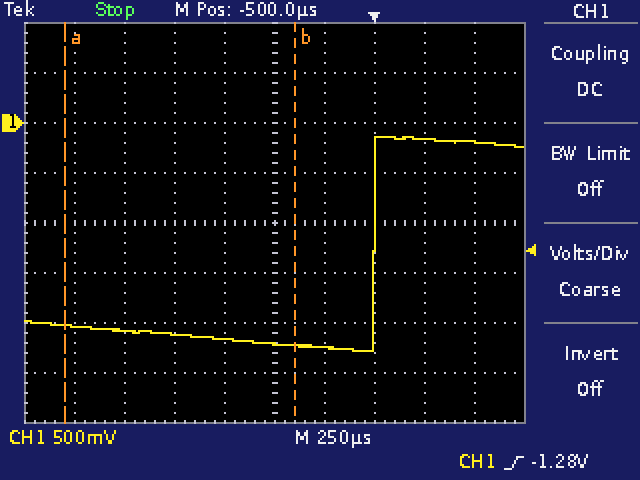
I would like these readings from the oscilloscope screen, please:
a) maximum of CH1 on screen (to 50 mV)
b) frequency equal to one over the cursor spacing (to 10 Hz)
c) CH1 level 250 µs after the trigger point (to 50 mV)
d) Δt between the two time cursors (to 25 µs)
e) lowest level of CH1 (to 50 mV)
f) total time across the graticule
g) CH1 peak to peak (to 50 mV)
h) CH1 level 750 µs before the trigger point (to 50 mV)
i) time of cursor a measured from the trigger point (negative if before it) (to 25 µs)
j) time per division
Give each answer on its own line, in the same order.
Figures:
-150 mV
870 Hz
-150 mV
1.150 ms
-2.30 V
2.5 ms
2.15 V
-2.15 V
-1.550 ms
250 µs
